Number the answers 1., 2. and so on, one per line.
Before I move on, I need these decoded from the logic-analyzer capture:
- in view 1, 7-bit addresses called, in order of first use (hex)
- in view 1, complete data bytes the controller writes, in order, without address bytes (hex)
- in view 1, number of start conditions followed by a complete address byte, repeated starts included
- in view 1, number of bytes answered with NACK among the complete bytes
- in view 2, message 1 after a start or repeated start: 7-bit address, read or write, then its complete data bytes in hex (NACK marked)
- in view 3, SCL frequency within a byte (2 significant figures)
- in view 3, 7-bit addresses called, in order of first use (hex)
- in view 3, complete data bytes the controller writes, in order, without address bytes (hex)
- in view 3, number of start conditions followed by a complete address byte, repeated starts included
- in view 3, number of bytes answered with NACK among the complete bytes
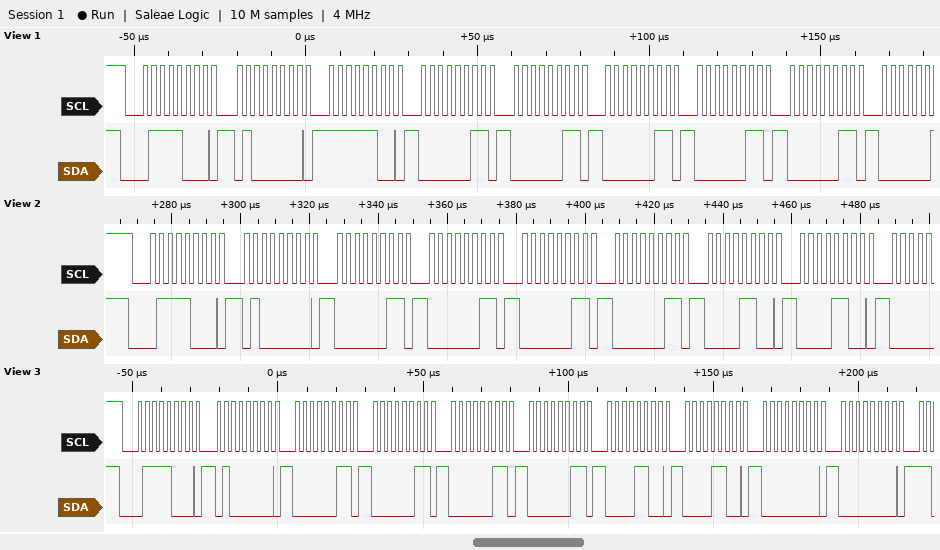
1. 0x3C
2. 40 FC 03 03 03 03 03
3. 1
4. 0
5. 0x3C write: 40 03 03 03 03 0C 0C
6. 400 kHz
7. 0x3C
8. 40 03 03 03 03 0C 0C 00 00
9. 1
10. 0
